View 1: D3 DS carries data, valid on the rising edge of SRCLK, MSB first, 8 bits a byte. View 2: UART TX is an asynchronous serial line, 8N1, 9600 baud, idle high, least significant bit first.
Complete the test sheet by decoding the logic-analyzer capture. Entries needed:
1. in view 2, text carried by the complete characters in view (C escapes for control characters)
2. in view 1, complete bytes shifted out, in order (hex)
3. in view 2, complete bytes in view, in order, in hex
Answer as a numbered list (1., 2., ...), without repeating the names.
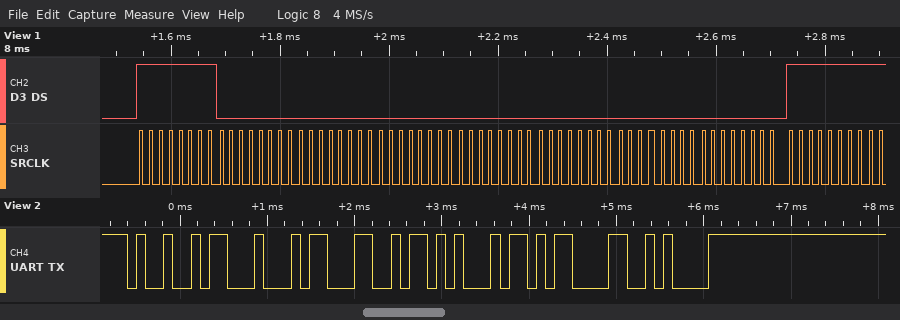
1. "IDLE\r\n"
2. FF 00 00 00 00 00 00 00 FF
3. 0x49 0x44 0x4C 0x45 0x0D 0x0A
